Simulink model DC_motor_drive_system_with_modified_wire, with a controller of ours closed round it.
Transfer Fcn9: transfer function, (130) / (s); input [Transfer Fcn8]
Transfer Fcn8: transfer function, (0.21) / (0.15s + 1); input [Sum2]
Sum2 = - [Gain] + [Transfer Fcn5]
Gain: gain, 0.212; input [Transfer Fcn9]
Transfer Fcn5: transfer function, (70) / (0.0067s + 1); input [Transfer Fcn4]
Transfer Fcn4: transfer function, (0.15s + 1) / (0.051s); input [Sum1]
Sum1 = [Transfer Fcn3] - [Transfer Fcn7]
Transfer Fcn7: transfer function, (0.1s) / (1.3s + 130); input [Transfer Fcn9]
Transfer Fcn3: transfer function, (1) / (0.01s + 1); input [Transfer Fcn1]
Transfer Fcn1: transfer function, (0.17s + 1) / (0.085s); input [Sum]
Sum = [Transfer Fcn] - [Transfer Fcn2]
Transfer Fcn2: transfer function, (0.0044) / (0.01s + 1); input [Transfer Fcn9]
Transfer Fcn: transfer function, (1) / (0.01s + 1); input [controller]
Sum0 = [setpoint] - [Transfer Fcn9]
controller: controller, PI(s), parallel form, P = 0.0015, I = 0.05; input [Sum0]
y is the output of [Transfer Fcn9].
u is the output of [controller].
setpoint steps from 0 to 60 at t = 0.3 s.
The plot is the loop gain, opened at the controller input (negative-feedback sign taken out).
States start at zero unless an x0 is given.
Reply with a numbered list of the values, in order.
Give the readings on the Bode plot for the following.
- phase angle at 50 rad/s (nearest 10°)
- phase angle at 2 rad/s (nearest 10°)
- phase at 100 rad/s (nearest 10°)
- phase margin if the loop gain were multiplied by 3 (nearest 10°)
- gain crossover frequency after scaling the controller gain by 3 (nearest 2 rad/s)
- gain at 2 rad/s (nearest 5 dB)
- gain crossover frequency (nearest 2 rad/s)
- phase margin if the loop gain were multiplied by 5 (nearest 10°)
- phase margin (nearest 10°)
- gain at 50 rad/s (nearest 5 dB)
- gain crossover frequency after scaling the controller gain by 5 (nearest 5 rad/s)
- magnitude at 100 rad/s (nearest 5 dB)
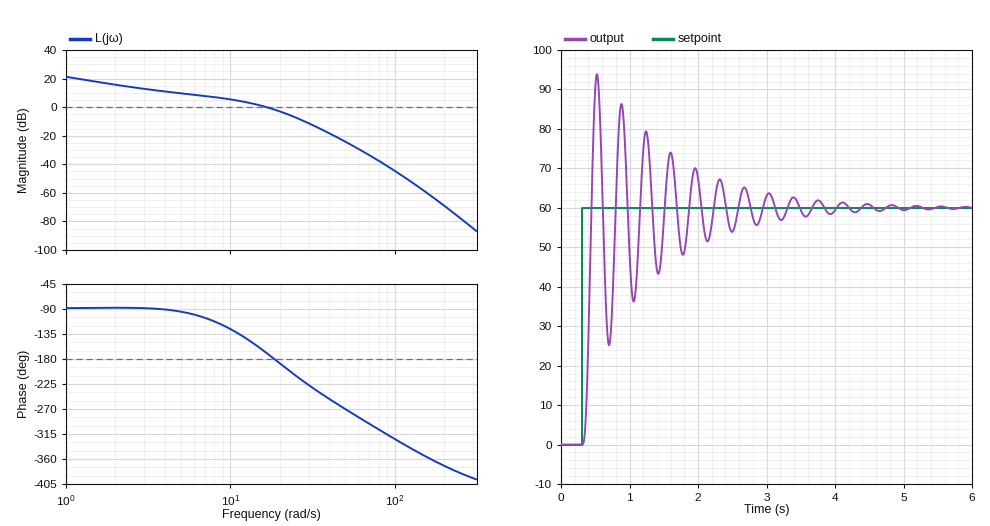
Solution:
1. -270°
2. -90°
3. -320°
4. -40°
5. 28 rad/s
6. 15 dB
7. 16 rad/s
8. -60°
9. 10°
10. -25 dB
11. 35 rad/s
12. -45 dB
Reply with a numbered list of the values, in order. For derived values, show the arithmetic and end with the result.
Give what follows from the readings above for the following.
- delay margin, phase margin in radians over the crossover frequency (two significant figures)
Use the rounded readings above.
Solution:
1. 10 × π / 180 / 16 = 0.011 s
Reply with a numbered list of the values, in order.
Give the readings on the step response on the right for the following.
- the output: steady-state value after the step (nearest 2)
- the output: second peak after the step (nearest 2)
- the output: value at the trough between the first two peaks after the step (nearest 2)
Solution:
1. 60
2. 86
3. 26
